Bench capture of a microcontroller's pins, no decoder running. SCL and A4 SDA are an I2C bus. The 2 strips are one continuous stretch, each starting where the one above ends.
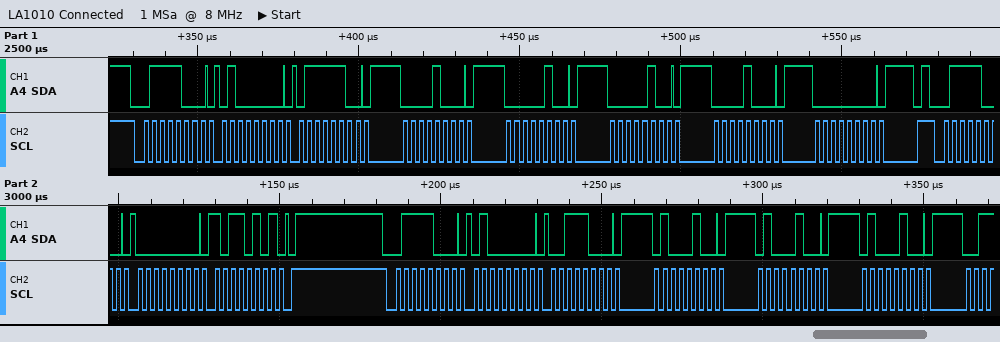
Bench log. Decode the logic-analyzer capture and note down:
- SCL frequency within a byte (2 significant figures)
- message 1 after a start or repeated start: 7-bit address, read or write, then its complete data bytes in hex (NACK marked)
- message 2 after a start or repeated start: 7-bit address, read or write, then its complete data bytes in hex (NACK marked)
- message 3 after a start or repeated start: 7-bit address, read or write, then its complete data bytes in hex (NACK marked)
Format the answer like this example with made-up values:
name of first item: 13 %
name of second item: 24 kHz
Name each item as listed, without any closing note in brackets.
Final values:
SCL frequency within a byte: 400 kHz
message 1 after a start or repeated start: 7-bit address, read or write, then its complete data bytes in hex: 0x3C write: 40 7C 08 04 04 08 00
message 2 after a start or repeated start: 7-bit address, read or write, then its complete data bytes in hex: 0x3C write: 00 B5
message 3 after a start or repeated start: 7-bit address, read or write, then its complete data bytes in hex: 0x3C write: 40 38 44 44 44
